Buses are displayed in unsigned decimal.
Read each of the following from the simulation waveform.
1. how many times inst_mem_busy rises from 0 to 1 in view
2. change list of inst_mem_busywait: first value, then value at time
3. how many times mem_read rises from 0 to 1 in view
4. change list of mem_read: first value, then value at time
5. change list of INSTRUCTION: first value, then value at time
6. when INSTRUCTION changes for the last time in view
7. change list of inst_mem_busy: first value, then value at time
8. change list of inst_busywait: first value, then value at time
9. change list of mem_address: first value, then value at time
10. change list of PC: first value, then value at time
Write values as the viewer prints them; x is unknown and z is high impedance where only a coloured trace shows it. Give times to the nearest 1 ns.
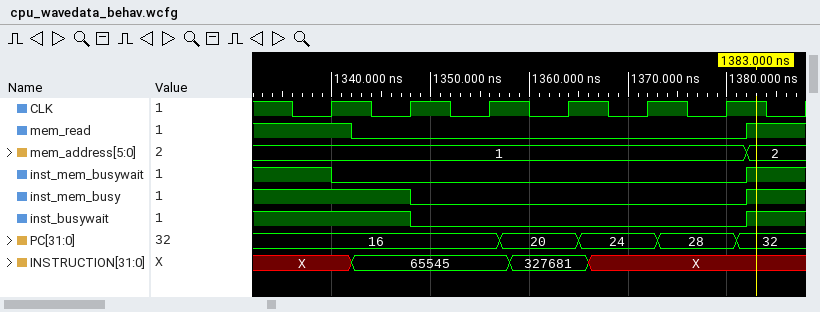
1
1, 0 at 1340 ns, 1 at 1382 ns
1
1, 0 at 1342 ns, 1 at 1382 ns
X, 65545 at 1342 ns, 327681 at 1358 ns, X at 1366 ns
1366 ns
1, 0 at 1348 ns, 1 at 1382 ns
1, 0 at 1348 ns, 1 at 1382 ns
1, 2 at 1382 ns
16, 20 at 1357 ns, 24 at 1365 ns, 28 at 1373 ns, 32 at 1381 ns
